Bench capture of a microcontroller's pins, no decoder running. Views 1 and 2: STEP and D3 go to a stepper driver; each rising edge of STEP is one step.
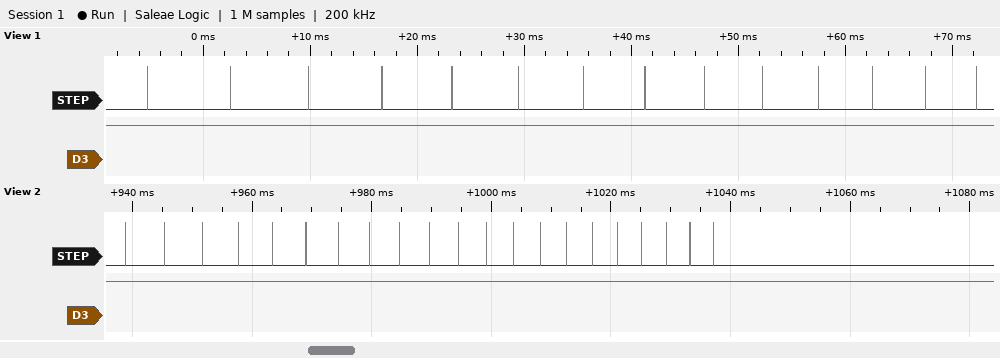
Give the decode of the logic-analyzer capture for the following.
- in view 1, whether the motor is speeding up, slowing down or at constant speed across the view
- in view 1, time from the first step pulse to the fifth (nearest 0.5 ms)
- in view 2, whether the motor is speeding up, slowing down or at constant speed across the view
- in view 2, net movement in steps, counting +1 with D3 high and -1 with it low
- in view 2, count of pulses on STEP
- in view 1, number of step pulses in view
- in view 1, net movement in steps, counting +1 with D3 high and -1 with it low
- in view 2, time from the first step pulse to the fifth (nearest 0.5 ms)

speeding up
28.5 ms
speeding up
+21
21
14
+14
24.5 ms
